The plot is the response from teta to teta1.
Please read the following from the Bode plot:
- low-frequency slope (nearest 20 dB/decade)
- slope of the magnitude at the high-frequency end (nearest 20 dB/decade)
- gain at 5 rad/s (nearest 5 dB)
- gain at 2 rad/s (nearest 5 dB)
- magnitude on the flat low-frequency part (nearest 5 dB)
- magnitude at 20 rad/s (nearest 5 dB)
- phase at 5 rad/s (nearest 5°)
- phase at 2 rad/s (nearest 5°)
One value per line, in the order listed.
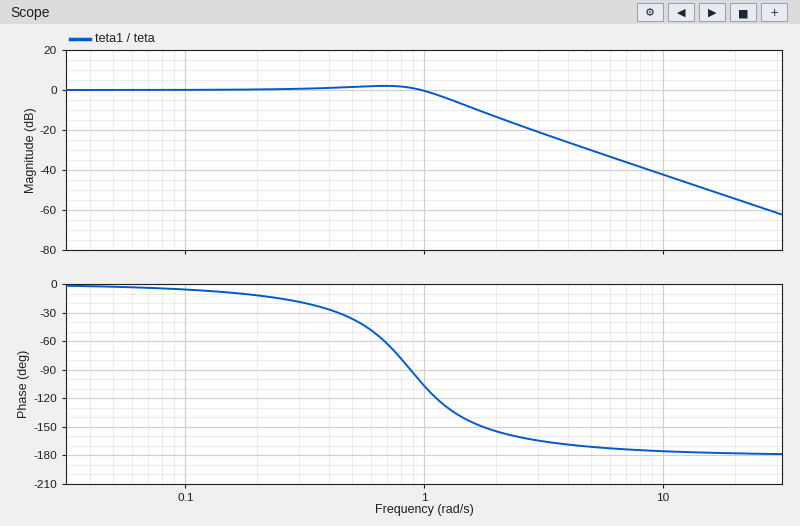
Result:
0 dB/decade
-40 dB/decade
-30 dB
-15 dB
0 dB
-55 dB
-170°
-155°
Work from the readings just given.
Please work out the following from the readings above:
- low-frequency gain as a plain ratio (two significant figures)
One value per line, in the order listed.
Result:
1.0
